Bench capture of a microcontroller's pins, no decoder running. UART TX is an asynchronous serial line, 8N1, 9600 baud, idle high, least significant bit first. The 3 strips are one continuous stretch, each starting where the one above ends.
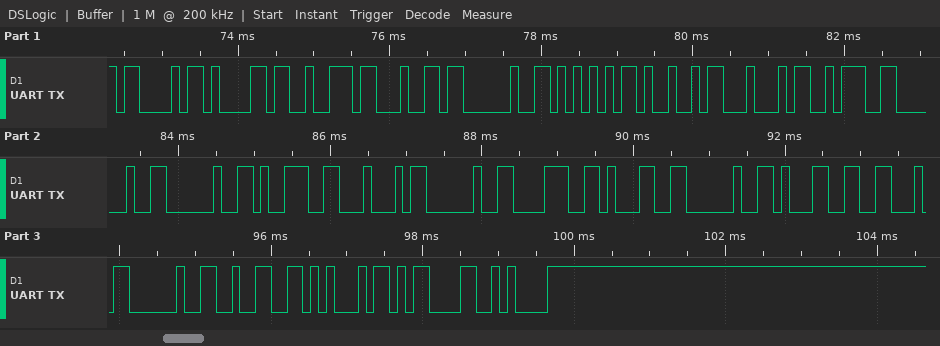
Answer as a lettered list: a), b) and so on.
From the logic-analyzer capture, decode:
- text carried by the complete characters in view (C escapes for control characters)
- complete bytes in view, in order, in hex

a) "Card UID:  9D 81 1F 2E\r\n"
b) 43 61 72 64 20 55 49 44 3A 20 20 39 44 20 38 31 20 31 46 20 32 45 0D 0A
